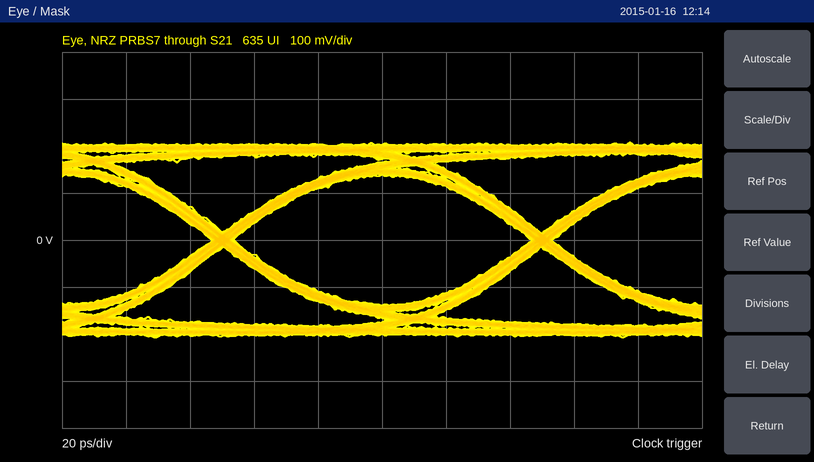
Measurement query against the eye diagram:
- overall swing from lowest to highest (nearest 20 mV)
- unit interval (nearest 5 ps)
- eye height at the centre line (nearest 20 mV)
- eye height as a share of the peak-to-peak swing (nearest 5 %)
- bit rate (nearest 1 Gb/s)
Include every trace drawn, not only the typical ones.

420 mV
100 ps
280 mV
65 %
10 Gb/s
